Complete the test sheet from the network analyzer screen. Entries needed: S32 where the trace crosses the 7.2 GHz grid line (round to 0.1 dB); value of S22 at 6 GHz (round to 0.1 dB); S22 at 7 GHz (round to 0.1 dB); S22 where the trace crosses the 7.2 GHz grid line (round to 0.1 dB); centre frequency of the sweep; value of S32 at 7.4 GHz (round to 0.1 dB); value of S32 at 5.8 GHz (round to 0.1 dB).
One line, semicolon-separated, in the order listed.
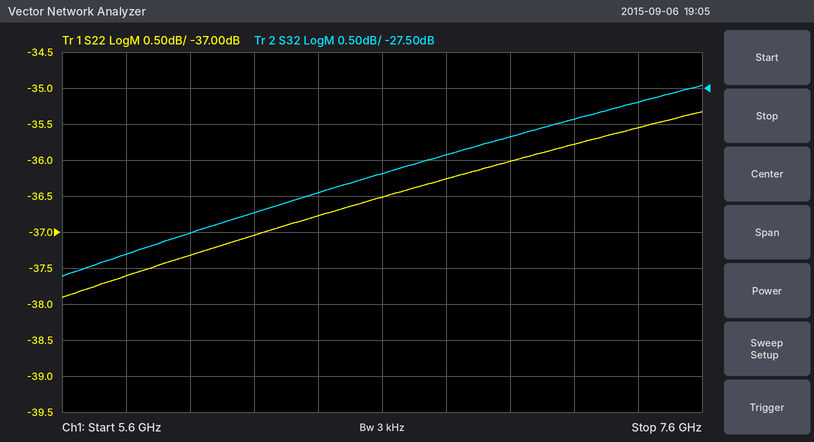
-27.9 dB; -37.3 dB; -36.0 dB; -35.8 dB; 6.6 GHz; -27.7 dB; -29.8 dB
